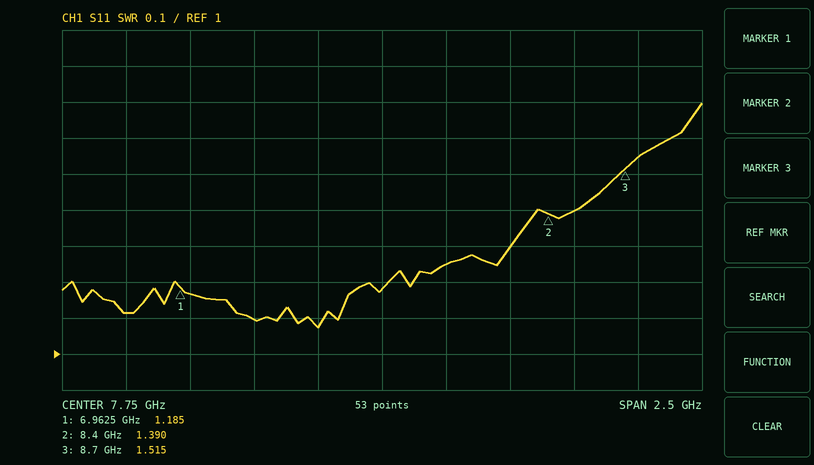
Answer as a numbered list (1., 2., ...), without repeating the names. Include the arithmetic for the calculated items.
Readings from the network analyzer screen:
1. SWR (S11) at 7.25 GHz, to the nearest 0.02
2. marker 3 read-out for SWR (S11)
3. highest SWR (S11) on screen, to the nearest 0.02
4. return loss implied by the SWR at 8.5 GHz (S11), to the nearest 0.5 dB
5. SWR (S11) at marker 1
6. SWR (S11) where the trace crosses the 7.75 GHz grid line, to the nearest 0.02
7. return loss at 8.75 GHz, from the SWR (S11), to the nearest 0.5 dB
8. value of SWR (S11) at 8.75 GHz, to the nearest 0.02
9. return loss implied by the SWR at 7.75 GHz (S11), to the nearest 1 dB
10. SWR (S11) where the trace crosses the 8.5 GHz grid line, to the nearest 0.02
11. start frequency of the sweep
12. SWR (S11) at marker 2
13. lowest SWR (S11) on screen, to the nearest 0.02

1. 1.10
2. 1.515
3. 1.70
4. −20 log10((1.4 − 1)/(1.4 + 1)) ≈ 15.6 dB, so 15.5 dB to the nearest 0.5 dB
5. 1.185
6. 1.18
7. −20 log10((1.54 − 1)/(1.54 + 1)) ≈ 13.4 dB, so 13.5 dB to the nearest 0.5 dB
8. 1.54
9. −20 log10((1.18 − 1)/(1.18 + 1)) ≈ 22 dB
10. 1.40
11. 6.5 GHz
12. 1.390
13. 1.08
